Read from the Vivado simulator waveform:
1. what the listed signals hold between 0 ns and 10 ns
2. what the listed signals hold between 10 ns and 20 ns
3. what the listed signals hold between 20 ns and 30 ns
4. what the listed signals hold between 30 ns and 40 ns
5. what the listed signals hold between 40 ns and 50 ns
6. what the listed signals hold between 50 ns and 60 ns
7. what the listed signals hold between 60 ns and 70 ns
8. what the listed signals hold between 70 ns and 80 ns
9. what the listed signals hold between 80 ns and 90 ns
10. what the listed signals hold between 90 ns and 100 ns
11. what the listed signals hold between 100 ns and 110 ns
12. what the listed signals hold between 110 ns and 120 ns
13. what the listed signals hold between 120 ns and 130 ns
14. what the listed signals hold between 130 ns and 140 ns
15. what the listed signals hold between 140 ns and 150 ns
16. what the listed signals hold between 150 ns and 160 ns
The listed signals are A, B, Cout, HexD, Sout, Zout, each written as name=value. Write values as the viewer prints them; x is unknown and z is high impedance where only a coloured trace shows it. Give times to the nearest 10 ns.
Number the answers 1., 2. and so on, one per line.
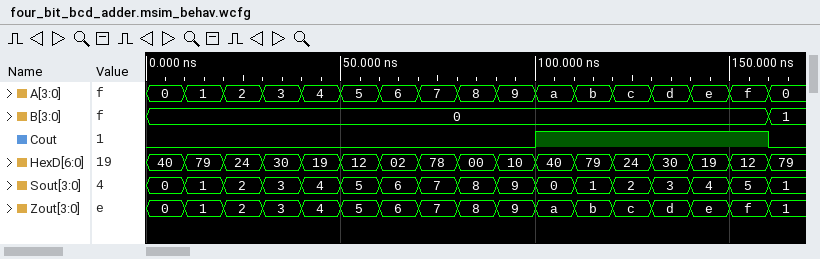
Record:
1. A=0, B=0, Cout=0, HexD=40, Sout=0, Zout=0
2. A=1, B=0, Cout=0, HexD=79, Sout=1, Zout=1
3. A=2, B=0, Cout=0, HexD=24, Sout=2, Zout=2
4. A=3, B=0, Cout=0, HexD=30, Sout=3, Zout=3
5. A=4, B=0, Cout=0, HexD=19, Sout=4, Zout=4
6. A=5, B=0, Cout=0, HexD=12, Sout=5, Zout=5
7. A=6, B=0, Cout=0, HexD=02, Sout=6, Zout=6
8. A=7, B=0, Cout=0, HexD=78, Sout=7, Zout=7
9. A=8, B=0, Cout=0, HexD=00, Sout=8, Zout=8
10. A=9, B=0, Cout=0, HexD=10, Sout=9, Zout=9
11. A=a, B=0, Cout=1, HexD=40, Sout=0, Zout=a
12. A=b, B=0, Cout=1, HexD=79, Sout=1, Zout=b
13. A=c, B=0, Cout=1, HexD=24, Sout=2, Zout=c
14. A=d, B=0, Cout=1, HexD=30, Sout=3, Zout=d
15. A=e, B=0, Cout=1, HexD=19, Sout=4, Zout=e
16. A=f, B=0, Cout=1, HexD=12, Sout=5, Zout=f
